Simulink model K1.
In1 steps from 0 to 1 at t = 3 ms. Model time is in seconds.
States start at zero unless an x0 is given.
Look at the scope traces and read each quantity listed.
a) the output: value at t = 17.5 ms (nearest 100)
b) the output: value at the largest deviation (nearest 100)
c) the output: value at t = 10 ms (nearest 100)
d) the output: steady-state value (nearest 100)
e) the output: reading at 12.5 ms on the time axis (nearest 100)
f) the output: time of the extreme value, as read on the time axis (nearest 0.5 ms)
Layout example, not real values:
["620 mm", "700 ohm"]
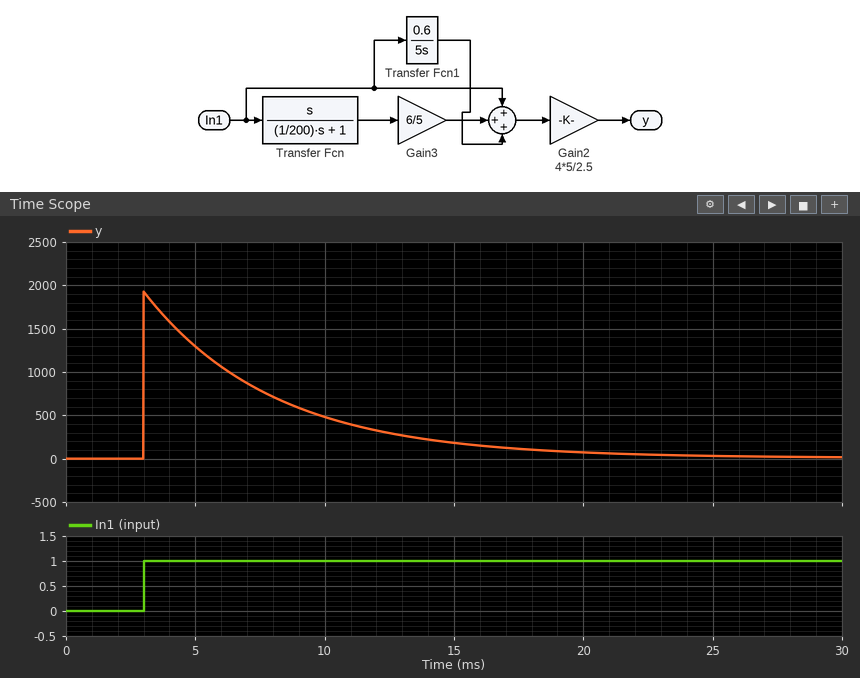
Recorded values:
["100", "1900", "500", "0", "300", "3.0 ms"]
